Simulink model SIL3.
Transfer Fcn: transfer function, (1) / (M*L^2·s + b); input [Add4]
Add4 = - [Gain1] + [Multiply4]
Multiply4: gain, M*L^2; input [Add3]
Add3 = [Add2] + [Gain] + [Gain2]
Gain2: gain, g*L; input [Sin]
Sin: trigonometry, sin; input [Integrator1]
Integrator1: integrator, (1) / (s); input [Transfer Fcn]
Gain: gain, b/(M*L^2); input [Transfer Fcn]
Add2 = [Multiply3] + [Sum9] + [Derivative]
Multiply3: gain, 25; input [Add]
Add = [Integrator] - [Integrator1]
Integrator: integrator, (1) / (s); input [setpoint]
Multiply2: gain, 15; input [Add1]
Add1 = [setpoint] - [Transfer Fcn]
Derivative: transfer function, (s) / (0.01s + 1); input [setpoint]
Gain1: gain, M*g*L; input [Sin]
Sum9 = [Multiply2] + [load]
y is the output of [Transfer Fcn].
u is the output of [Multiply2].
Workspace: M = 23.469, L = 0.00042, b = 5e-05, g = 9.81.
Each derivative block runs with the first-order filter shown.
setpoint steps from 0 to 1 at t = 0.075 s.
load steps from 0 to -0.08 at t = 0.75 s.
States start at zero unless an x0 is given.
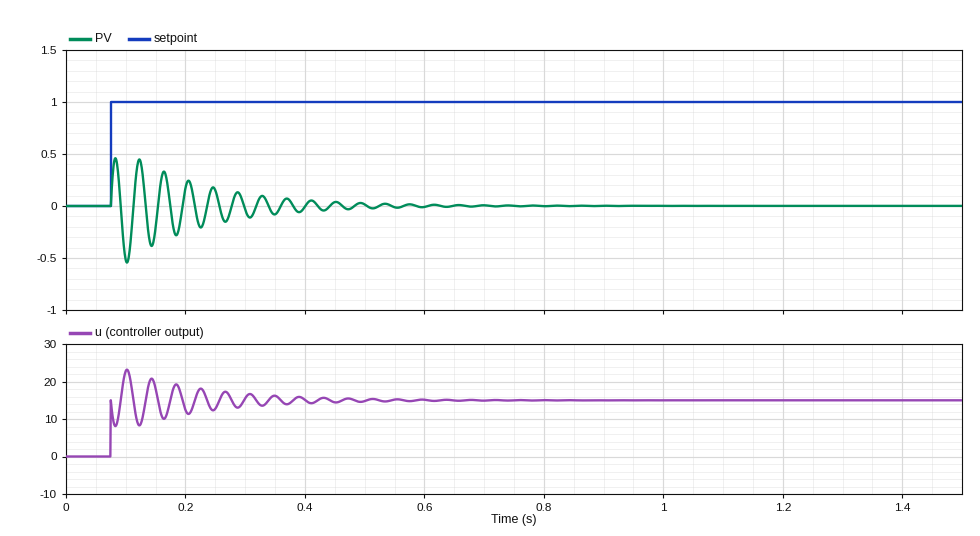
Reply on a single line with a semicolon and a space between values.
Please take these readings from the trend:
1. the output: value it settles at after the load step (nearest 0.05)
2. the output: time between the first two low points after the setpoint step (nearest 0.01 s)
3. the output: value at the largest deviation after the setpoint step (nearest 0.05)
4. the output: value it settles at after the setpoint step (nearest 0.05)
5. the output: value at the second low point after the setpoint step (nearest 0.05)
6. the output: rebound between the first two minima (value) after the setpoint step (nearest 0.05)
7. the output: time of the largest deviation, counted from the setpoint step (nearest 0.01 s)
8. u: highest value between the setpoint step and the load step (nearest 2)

0.00; 0.04 s; -0.55; 0.00; -0.40; 0.45; 0.03 s; 24
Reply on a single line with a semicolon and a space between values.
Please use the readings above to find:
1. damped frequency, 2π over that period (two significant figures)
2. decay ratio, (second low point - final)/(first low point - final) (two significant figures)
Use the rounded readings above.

160 rad/s; 0.73
